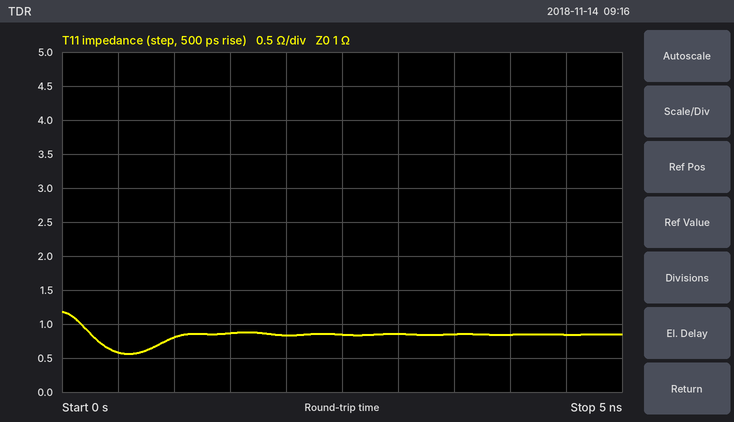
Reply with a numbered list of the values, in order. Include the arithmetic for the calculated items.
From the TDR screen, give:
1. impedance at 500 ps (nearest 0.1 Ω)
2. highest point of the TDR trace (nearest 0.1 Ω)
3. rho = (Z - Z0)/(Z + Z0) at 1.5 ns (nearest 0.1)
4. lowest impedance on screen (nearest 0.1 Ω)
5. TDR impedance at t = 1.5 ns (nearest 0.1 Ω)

1. 0.6 Ω
2. 1.2 Ω
3. (0.9 − 1)/(0.9 + 1) ≈ -0.1
4. 0.6 Ω
5. 0.9 Ω
